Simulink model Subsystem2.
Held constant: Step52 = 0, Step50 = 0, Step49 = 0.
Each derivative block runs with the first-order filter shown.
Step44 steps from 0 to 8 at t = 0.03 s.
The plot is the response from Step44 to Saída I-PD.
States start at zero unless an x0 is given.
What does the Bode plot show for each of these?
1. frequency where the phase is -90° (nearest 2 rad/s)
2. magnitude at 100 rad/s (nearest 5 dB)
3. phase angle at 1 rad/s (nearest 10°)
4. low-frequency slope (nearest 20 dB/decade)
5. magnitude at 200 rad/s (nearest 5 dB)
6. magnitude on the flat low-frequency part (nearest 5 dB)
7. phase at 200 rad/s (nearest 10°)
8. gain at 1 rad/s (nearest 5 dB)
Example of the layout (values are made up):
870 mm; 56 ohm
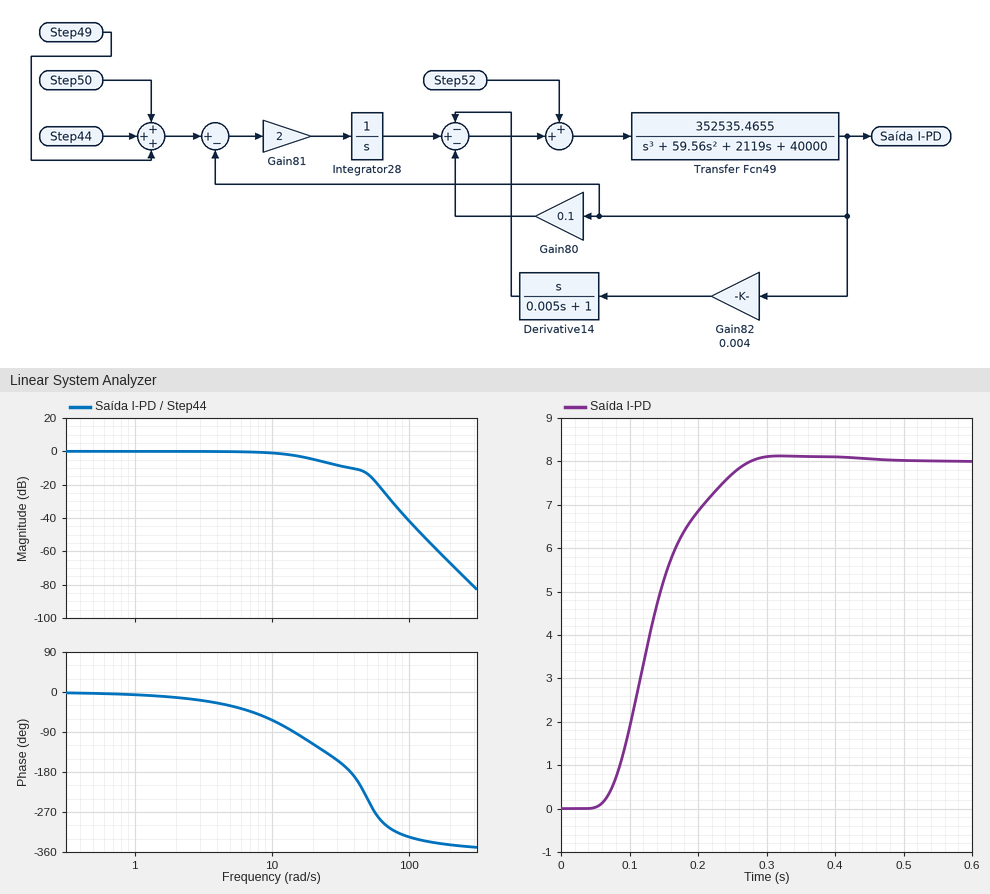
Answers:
14 rad/s; -40 dB; -10°; 0 dB/decade; -65 dB; 0 dB; -340°; 0 dB
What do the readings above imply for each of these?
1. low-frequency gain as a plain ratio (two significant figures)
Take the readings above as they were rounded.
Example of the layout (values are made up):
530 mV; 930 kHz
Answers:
1.0
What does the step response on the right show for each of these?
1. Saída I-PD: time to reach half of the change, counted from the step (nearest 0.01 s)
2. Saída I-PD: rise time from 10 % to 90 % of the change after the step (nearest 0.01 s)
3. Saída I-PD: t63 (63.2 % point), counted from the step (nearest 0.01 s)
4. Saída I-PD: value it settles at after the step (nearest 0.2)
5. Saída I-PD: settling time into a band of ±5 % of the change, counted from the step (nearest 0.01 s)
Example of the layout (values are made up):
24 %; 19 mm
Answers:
0.10 s; 0.14 s; 0.12 s; 8.0; 0.21 s
